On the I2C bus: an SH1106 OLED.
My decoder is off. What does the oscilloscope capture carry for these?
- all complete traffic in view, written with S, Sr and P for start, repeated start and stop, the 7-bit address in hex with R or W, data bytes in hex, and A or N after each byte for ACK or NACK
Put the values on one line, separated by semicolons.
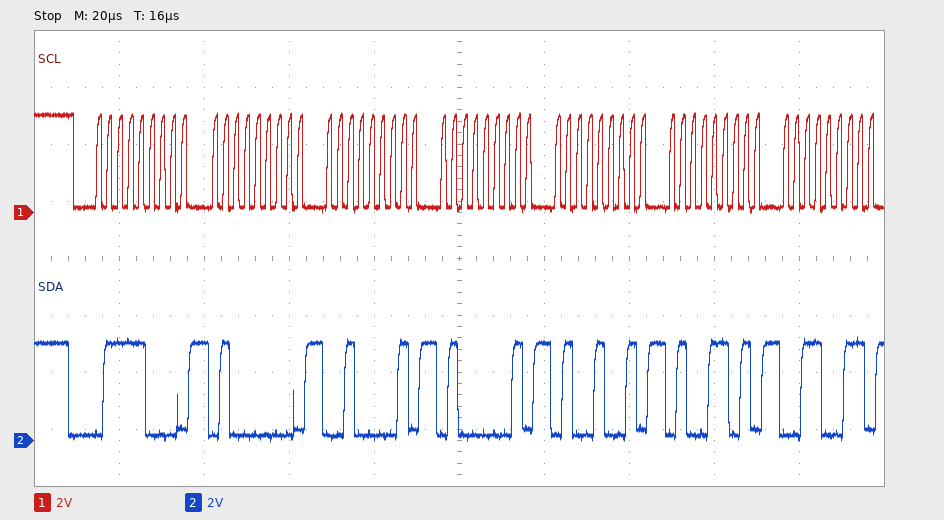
S 3CW A 40 A 21 A 41 A 49 A 4D A 33 A
